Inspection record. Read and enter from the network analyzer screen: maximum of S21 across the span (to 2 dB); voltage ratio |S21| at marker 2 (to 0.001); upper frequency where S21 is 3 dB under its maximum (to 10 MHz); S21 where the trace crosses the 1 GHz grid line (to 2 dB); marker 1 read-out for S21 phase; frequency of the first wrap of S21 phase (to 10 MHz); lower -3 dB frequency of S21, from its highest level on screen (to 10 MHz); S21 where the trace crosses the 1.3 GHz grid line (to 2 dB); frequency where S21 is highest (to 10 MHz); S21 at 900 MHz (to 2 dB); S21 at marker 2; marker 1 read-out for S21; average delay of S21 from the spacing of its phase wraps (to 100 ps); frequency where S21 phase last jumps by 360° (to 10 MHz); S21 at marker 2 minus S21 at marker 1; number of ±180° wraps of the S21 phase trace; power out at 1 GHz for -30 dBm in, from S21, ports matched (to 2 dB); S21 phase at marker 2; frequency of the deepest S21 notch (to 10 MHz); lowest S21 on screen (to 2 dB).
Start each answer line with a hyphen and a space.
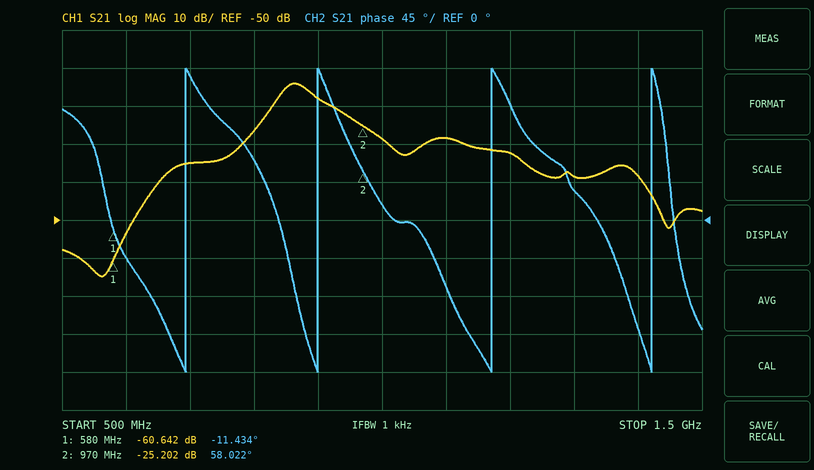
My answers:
- -14 dB
- 0.055
- 890 MHz
- -28 dB
- -11.434°
- 690 MHz
- 840 MHz
- -38 dB
- 860 MHz
- -18 dB
- -25.202 dB
- -60.642 dB
- 4.1 ns
- 1.42 GHz
- 35.440 dB
- 4
- -58 dBm
- 58.022°
- 560 MHz
- -64 dB
